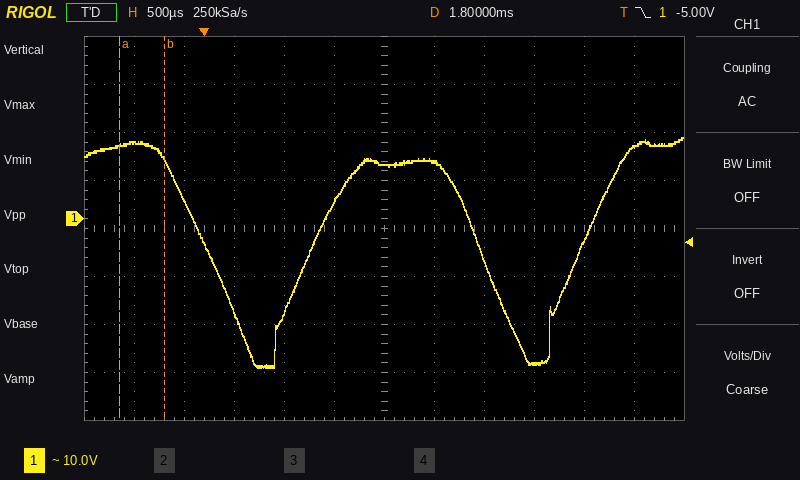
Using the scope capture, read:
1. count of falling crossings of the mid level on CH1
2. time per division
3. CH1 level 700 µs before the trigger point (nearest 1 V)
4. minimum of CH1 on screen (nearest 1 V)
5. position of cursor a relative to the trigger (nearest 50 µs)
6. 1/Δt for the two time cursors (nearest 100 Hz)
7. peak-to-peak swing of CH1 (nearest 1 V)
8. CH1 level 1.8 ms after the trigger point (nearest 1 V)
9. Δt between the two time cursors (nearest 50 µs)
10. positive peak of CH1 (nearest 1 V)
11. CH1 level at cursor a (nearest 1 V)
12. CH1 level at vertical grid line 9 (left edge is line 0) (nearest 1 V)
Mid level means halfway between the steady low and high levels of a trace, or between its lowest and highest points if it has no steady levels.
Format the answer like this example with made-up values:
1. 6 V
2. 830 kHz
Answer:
1. 2
2. 500 µs
3. 16 V
4. -31 V
5. -850 µs
6. 2.2 kHz
7. 48 V
8. 11 V
9. 450 µs
10. 17 V
11. 15 V
12. -30 V
